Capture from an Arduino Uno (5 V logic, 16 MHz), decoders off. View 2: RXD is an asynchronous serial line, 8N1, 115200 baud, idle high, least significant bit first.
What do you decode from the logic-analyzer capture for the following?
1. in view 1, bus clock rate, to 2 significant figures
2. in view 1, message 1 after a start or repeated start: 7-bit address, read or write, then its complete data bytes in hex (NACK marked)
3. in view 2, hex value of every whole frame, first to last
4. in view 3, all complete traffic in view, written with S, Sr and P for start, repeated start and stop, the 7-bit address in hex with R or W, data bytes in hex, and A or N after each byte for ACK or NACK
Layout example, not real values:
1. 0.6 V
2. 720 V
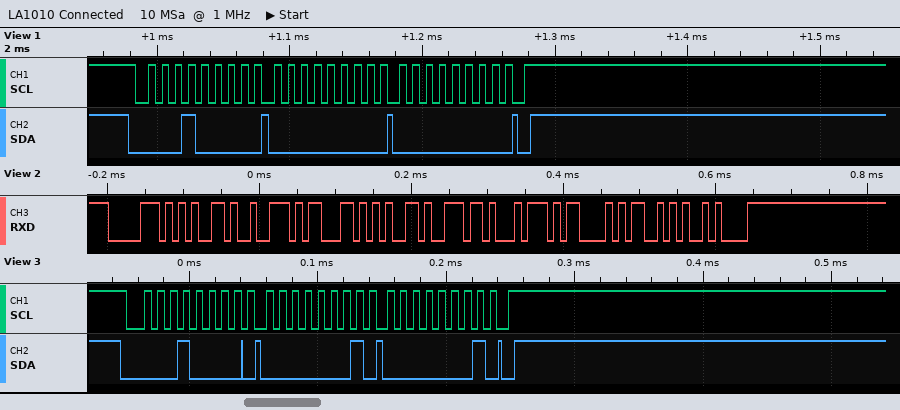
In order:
1. 100 kHz
2. 0x08 write: 00 00
3. 70 65 72 63 65 6E 74 43 53 0A
4. S 08W A 01 A 01 A P
